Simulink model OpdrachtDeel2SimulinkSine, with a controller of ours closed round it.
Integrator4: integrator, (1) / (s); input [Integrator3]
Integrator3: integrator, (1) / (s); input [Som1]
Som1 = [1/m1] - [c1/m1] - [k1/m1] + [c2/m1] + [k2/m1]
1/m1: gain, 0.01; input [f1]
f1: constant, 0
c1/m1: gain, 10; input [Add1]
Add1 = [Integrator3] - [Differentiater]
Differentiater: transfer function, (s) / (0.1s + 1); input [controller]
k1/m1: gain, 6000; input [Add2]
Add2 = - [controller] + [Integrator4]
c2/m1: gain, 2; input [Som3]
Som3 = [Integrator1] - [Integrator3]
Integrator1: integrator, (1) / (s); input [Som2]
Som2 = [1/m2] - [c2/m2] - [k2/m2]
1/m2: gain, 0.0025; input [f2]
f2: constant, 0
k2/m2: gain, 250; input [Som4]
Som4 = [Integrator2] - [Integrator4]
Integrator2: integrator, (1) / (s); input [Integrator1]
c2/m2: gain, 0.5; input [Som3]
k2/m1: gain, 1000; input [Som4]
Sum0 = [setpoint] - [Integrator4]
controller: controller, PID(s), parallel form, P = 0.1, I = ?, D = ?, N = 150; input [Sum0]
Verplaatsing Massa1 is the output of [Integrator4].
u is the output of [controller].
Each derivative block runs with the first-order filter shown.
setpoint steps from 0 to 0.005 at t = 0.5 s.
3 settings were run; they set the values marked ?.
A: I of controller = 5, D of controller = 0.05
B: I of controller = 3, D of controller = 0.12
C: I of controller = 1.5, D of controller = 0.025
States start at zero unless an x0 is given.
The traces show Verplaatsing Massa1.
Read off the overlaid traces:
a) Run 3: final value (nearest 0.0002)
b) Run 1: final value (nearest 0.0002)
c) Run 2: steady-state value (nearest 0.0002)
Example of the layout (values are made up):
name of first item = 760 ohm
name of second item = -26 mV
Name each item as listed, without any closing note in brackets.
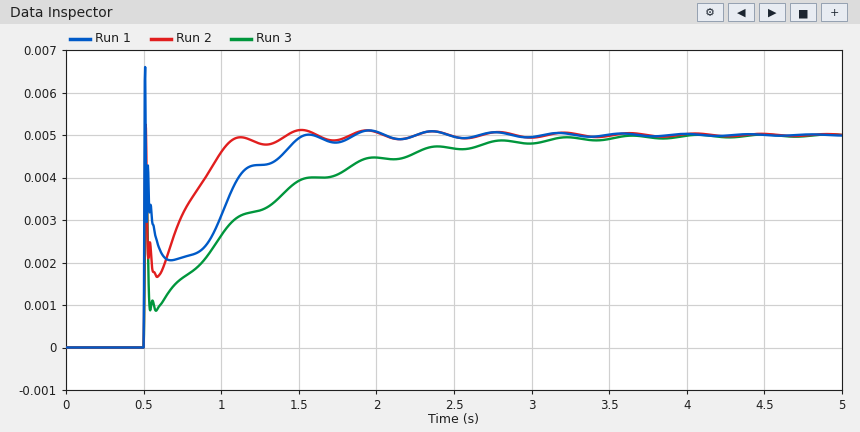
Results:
Run 3: final value = 0.0050
Run 1: final value = 0.0050
Run 2: steady-state value = 0.0050
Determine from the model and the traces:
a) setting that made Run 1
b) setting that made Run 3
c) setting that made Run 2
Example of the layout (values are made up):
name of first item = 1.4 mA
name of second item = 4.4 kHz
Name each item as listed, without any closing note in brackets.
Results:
setting that made Run 1 = B
setting that made Run 3 = C
setting that made Run 2 = A
